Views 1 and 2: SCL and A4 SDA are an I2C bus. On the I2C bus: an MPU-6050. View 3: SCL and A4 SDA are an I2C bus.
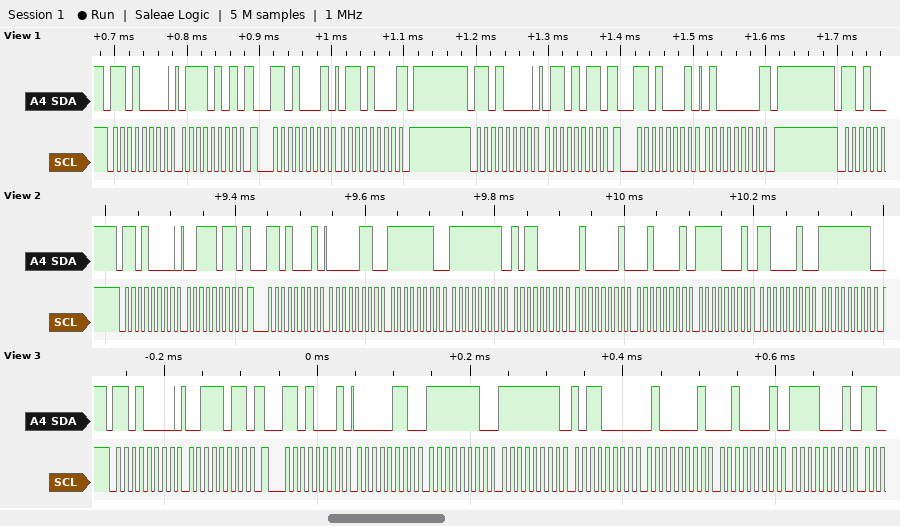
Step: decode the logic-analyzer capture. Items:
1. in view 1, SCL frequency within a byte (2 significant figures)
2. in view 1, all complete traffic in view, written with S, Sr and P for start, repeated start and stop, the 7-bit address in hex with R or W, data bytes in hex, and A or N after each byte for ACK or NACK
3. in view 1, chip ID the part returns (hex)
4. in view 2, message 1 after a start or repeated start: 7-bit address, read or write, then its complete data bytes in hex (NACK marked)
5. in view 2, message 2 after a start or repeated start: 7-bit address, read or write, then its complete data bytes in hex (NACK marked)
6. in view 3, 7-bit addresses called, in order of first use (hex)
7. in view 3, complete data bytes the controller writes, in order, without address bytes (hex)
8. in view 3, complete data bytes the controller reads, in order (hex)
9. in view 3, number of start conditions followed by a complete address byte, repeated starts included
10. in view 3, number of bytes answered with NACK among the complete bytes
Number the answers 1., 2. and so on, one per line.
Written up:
1. 100 kHz
2. S 68W A 75 A Sr 68R A 68 N P S 68W A 6B A Sr 68R A 40 N P
3. 0x68
4. 0x68 write: 3B
5. 0x68 read: 06 FE FF B0 41 21 F1 C2 FF
6. 0x68
7. 3B
8. 06 FE FF B0 41 21 F1
9. 2
10. 0
